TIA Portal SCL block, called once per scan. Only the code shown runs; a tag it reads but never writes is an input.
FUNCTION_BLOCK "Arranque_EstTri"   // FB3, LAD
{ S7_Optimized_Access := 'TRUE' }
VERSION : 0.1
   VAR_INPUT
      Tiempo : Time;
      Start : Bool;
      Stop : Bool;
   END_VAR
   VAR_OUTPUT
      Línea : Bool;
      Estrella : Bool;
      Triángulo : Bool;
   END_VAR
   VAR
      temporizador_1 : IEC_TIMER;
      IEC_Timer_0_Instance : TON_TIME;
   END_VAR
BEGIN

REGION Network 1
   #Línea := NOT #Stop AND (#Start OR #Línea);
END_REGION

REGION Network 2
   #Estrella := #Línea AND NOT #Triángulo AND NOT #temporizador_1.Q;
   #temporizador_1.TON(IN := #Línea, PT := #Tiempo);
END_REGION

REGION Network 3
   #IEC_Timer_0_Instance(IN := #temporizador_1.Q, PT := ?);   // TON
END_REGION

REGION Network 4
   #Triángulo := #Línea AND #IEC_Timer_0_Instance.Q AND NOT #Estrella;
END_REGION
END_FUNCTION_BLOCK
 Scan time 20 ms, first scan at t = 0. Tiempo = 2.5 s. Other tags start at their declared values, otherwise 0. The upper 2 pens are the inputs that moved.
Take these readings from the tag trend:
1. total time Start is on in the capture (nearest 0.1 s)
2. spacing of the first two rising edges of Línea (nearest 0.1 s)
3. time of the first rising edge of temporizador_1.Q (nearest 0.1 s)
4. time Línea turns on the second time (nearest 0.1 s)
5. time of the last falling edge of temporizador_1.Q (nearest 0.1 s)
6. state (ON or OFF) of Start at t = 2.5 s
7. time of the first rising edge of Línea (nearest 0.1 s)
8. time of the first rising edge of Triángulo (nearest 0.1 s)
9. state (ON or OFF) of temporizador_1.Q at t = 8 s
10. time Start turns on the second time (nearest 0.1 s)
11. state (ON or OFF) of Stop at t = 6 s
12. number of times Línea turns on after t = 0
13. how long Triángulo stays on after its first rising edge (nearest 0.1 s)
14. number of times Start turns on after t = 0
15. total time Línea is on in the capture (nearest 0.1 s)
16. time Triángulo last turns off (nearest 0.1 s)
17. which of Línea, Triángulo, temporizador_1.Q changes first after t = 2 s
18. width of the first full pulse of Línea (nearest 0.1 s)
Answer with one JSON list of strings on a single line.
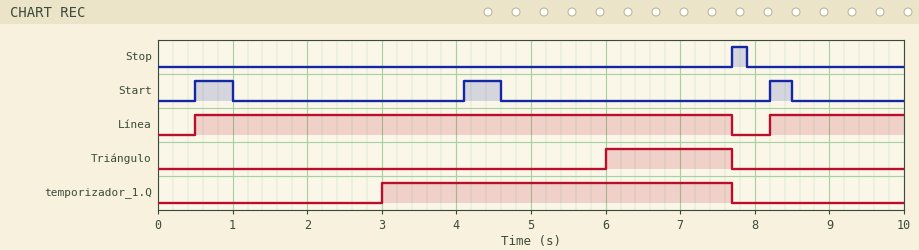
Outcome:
["1.3 s", "7.7 s", "3.0 s", "8.2 s", "7.7 s", "OFF", "0.5 s", "6.0 s", "OFF", "4.1 s", "OFF", "2", "1.7 s", "3", "9.0 s", "7.7 s", "temporizador_1.Q", "7.2 s"]
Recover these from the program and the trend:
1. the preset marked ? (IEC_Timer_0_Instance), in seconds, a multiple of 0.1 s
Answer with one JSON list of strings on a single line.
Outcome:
["3.0 s"]
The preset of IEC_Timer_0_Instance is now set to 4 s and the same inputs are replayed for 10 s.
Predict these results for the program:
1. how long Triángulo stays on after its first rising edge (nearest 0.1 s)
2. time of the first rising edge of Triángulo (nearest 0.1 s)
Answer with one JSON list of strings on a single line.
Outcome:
["0.7 s", "7.0 s"]
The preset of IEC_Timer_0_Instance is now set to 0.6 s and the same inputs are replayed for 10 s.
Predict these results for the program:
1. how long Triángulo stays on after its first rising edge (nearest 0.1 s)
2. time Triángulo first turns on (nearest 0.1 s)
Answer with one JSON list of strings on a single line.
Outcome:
["4.1 s", "3.6 s"]
